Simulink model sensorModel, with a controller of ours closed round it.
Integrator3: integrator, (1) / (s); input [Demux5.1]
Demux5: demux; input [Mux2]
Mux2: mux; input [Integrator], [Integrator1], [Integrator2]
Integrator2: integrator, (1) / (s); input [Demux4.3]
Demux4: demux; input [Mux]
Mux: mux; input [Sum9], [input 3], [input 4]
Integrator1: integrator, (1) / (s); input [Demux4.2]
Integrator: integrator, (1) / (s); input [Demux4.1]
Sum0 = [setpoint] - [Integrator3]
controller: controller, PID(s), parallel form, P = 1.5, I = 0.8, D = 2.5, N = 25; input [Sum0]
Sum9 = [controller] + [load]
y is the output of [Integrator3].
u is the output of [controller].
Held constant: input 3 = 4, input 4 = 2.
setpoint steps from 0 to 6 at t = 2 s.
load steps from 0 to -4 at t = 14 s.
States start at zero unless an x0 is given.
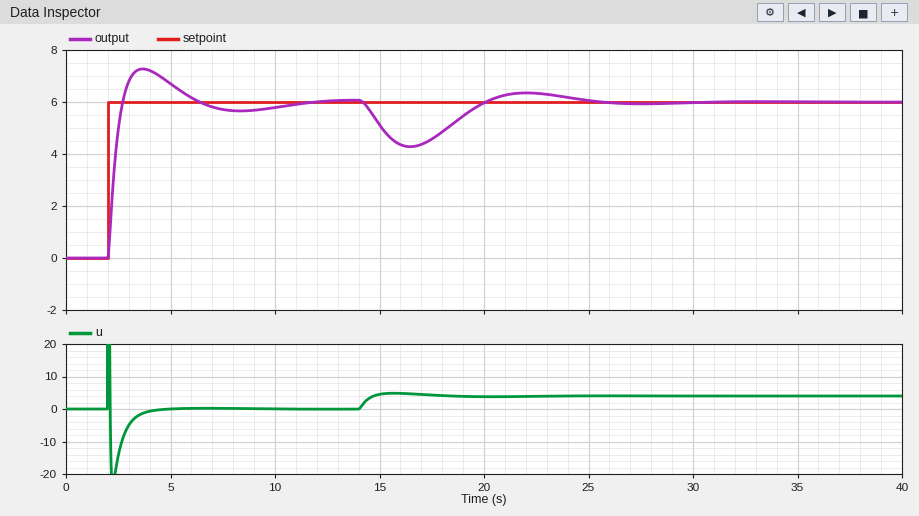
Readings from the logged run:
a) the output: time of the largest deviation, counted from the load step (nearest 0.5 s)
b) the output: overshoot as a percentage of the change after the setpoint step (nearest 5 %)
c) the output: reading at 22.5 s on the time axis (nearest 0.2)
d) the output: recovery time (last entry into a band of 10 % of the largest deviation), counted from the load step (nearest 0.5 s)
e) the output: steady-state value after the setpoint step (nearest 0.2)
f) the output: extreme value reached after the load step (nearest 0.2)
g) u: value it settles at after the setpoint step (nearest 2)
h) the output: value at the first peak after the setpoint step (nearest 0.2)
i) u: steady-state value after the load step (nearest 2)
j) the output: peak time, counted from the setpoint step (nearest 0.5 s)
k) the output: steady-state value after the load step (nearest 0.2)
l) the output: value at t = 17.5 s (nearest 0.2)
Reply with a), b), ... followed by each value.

a) 2.5 s
b) 20 %
c) 6.4
d) 10.0 s
e) 6.0
f) 4.2
g) 0
h) 7.2
i) 4
j) 1.5 s
k) 6.0
l) 4.6
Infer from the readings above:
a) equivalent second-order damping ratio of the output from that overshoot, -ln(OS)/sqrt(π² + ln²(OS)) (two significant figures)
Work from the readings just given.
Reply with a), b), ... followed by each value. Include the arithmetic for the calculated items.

a) ln(0.2) = -1.609; 1.609 / sqrt(9.870 + 2.590) = 0.46
